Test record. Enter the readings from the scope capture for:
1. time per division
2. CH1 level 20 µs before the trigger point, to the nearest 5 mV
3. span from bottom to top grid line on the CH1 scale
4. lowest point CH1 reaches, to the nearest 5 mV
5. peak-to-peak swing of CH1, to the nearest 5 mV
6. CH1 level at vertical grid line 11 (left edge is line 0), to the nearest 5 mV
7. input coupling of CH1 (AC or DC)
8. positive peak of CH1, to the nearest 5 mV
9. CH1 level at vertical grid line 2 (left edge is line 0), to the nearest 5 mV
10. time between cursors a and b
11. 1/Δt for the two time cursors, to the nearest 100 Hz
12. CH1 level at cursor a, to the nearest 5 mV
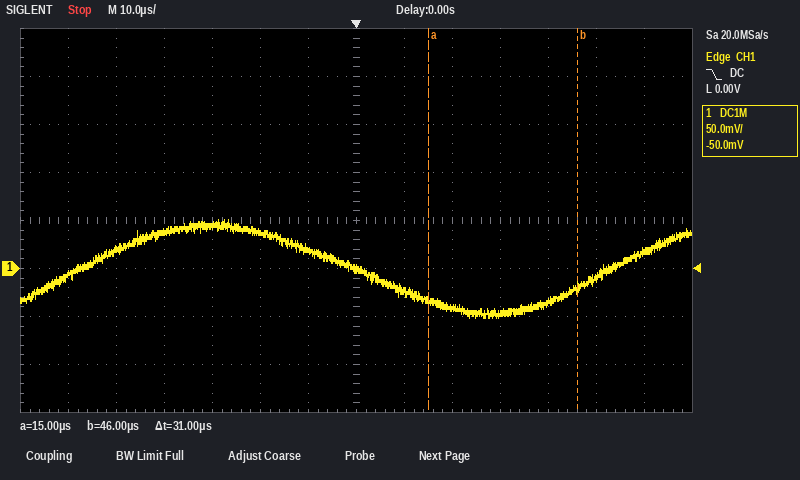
10 µs
40 mV
400 mV
-50 mV
100 mV
-35 mV
DC
50 mV
20 mV
31 µs
32.3 kHz
-35 mV
